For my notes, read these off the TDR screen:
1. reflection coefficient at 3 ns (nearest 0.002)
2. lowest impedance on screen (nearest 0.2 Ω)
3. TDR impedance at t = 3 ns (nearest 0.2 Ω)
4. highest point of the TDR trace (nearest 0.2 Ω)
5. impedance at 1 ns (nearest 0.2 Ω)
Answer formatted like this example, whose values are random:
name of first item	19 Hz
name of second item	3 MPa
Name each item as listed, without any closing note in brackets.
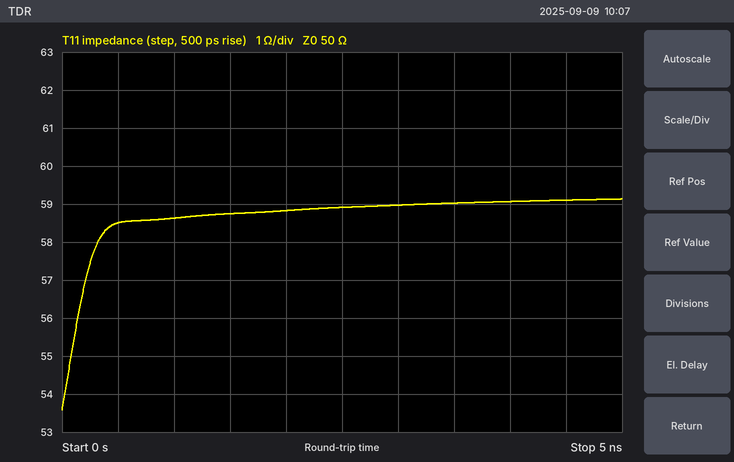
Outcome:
reflection coefficient at 3 ns	+0.082
lowest impedance on screen	53.6 Ω
TDR impedance at t = 3 ns	59.0 Ω
highest point of the TDR trace	59.2 Ω
impedance at 1 ns	58.6 Ω
